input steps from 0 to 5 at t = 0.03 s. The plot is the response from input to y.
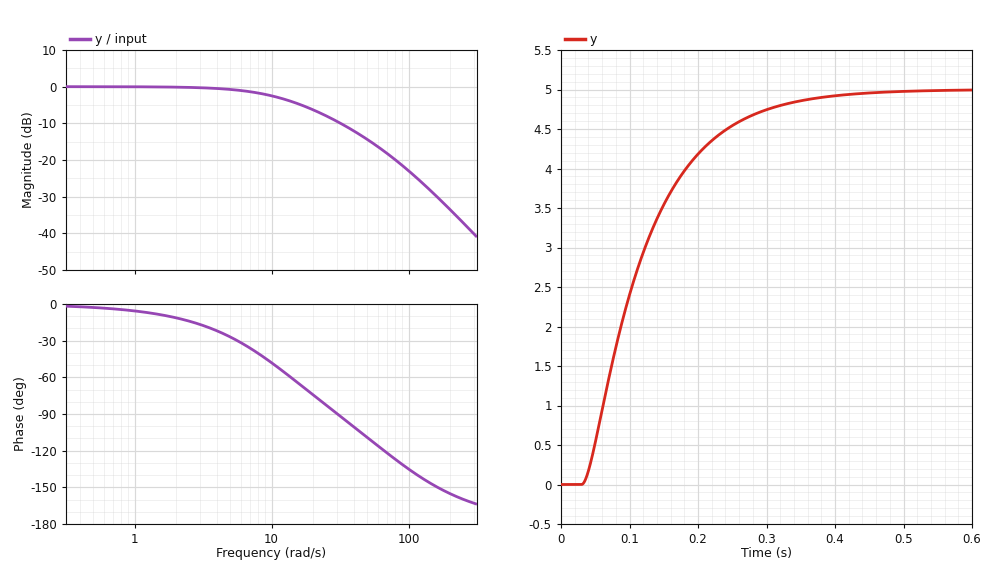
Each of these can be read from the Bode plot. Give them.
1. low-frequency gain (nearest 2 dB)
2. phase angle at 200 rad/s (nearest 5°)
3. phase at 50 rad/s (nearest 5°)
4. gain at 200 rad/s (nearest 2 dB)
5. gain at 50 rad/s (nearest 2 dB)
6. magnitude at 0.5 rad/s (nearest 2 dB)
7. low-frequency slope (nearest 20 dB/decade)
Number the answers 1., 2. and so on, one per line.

1. 0 dB
2. -155°
3. -110°
4. -34 dB
5. -14 dB
6. 0 dB
7. 0 dB/decade
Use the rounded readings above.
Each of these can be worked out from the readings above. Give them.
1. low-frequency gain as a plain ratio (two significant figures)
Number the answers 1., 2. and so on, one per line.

1. 1.0
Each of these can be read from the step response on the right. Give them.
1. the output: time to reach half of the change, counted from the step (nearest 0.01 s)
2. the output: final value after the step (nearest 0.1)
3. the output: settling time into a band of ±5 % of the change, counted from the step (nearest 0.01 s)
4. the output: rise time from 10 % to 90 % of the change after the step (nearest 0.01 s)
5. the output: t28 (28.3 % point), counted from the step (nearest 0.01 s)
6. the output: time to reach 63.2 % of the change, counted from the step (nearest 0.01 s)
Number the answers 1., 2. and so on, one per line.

1. 0.07 s
2. 5.0
3. 0.27 s
4. 0.19 s
5. 0.04 s
6. 0.10 s
